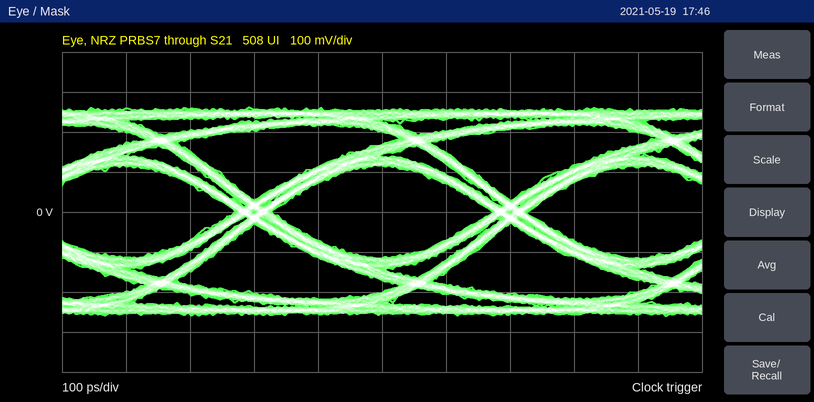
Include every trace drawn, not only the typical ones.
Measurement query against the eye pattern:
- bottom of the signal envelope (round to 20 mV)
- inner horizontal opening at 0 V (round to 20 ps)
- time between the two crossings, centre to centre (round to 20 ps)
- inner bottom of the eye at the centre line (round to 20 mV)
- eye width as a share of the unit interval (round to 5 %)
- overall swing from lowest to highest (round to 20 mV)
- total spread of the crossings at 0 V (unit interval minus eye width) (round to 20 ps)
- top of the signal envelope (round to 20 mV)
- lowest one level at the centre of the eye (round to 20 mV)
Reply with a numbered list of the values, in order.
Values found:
1. -260 mV
2. 340 ps
3. 400 ps
4. -120 mV
5. 85 %
6. 520 mV
7. 60 ps
8. 260 mV
9. 120 mV
